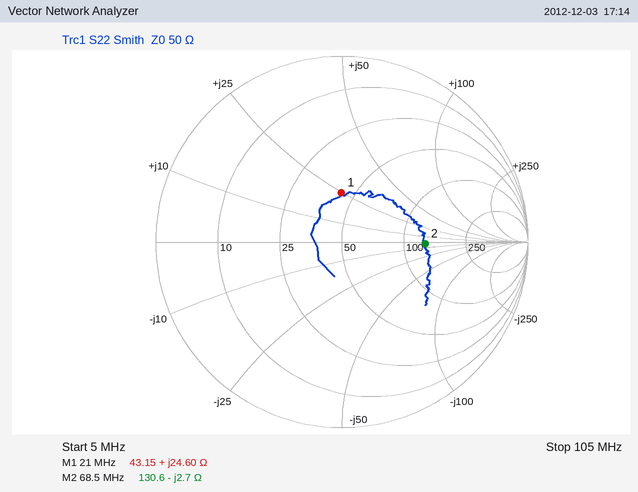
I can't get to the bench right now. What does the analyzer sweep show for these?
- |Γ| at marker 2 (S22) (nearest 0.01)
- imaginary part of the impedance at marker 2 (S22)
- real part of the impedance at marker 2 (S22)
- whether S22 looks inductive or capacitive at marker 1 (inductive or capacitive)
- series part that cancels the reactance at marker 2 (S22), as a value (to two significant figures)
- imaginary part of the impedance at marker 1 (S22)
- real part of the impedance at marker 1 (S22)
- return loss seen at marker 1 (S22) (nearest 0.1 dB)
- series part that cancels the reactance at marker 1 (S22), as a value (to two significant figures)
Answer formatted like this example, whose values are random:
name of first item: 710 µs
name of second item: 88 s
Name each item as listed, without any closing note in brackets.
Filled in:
|Γ| at marker 2 (S22): 0.45
imaginary part of the impedance at marker 2: -2.7 Ω
real part of the impedance at marker 2: 130.6 Ω
whether S22 looks inductive or capacitive at marker 1: inductive
series part that cancels the reactance at marker 2 (S22), as a value: 6.3 nH
imaginary part of the impedance at marker 1: +24.60 Ω
real part of the impedance at marker 1: 43.15 Ω
return loss seen at marker 1 (S22): 11.5 dB
series part that cancels the reactance at marker 1 (S22), as a value: 310 pF
